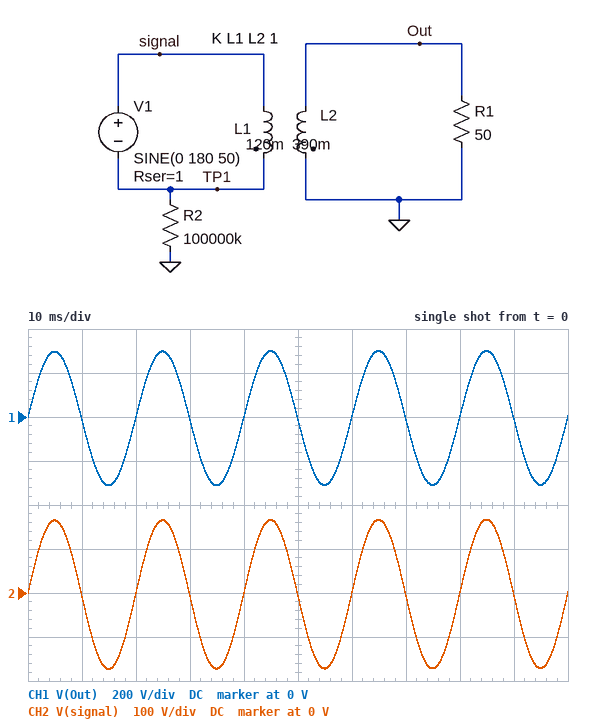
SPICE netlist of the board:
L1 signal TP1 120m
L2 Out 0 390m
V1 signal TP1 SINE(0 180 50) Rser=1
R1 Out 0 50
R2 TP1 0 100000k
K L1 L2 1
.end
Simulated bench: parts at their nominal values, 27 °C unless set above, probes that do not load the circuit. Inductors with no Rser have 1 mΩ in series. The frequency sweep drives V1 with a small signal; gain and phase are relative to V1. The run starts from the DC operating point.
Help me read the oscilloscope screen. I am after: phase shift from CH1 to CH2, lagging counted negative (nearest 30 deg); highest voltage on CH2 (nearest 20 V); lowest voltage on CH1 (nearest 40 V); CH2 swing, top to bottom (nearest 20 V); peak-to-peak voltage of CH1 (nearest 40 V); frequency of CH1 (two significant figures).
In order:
0 deg
160 V
-320 V
340 V
600 V
50 Hz
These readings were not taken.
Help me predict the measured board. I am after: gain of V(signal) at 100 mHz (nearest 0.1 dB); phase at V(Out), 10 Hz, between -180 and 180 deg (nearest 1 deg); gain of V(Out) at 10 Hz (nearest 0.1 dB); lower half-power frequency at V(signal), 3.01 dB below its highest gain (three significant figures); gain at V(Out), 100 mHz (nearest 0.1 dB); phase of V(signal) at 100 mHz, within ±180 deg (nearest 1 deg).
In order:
-22.5 dB
7 deg
4.5 dB
1.25 Hz
-17.4 dB
85 deg
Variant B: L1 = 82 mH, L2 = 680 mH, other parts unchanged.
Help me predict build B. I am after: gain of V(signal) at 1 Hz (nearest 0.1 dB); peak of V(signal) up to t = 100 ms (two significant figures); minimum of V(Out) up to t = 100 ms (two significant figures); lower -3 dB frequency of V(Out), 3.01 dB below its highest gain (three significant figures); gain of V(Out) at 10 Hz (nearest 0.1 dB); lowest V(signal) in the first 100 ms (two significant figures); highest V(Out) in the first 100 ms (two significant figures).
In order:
-7.1 dB
150 V
-460 V
1.67 Hz
7.7 dB
-160 V
440 V
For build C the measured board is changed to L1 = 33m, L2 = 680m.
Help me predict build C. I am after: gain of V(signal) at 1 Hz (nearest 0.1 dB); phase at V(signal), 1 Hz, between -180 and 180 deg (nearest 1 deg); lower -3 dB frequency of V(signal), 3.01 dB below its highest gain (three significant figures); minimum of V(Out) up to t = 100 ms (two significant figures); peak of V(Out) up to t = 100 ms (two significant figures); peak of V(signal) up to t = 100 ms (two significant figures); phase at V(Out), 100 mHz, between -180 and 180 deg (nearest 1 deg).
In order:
-14.0 dB
73 deg
3.42 Hz
-610 V
570 V
130 V
88 deg
